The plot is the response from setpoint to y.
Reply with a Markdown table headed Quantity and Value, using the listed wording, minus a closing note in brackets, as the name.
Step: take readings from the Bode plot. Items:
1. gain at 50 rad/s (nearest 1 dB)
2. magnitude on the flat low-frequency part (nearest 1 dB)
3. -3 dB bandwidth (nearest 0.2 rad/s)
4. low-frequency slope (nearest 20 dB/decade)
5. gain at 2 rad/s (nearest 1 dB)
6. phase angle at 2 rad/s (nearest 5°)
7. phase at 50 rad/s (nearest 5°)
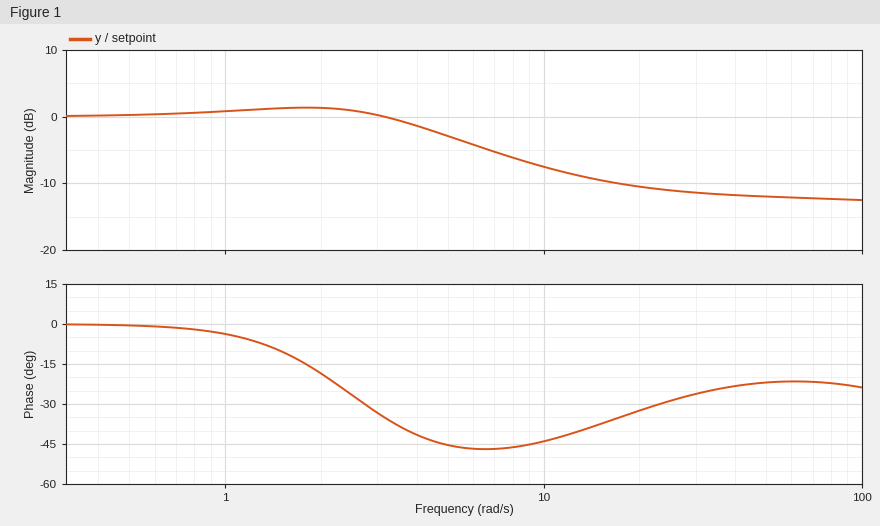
| Quantity | Value |
|---|---|
| gain at 50 rad/s | -12 dB |
| magnitude on the flat low-frequency part | 0 dB |
| -3 dB bandwidth | 5.0 rad/s |
| low-frequency slope | 0 dB/decade |
| gain at 2 rad/s | 1 dB |
| phase angle at 2 rad/s | -20° |
| phase at 50 rad/s | -20° |
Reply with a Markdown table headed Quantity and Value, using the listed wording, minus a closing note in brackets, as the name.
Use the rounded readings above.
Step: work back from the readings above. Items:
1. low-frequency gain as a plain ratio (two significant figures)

| Quantity | Value |
|---|---|
| low-frequency gain as a plain ratio | 1.0 |
